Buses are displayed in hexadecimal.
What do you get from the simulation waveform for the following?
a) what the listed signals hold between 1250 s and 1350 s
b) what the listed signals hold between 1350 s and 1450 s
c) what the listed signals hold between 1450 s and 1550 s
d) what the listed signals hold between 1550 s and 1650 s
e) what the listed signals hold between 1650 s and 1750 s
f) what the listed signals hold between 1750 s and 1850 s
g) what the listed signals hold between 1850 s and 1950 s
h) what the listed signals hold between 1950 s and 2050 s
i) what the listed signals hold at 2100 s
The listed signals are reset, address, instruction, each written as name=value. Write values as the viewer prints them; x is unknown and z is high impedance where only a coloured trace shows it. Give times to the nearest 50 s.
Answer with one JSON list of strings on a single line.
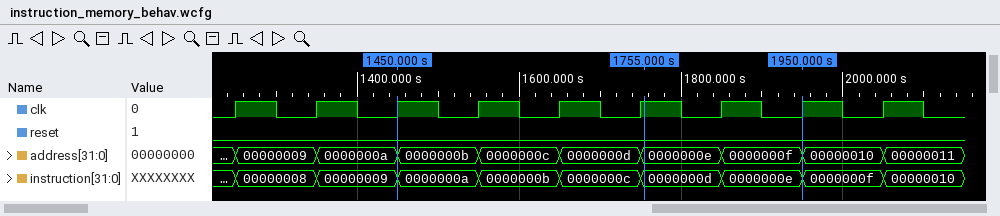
["reset=0, address=00000009, instruction=00000008", "reset=0, address=0000000a, instruction=00000009", "reset=0, address=0000000b, instruction=0000000a", "reset=0, address=0000000c, instruction=0000000b", "reset=0, address=0000000d, instruction=0000000c", "reset=0, address=0000000e, instruction=0000000d", "reset=0, address=0000000f, instruction=0000000e", "reset=0, address=00000010, instruction=0000000f", "reset=0, address=00000011, instruction=00000010"]
